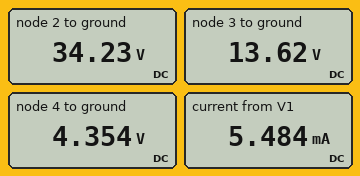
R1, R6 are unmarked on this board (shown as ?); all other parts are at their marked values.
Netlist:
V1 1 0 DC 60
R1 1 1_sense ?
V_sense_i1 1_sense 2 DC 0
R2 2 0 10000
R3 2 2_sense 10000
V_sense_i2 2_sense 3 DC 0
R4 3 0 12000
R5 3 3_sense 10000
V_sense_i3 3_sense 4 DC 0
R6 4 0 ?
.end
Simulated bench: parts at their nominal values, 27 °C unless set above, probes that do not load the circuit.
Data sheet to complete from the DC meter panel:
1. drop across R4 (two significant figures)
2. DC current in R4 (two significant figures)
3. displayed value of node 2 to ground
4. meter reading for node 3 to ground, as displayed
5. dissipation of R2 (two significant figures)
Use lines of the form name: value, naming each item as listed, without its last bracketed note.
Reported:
drop across R4: 14 V
DC current in R4: 1.1 mA
displayed value of node 2 to ground: 34.23 V
meter reading for node 3 to ground, as displayed: 13.62 V
dissipation of R2: 120 mW
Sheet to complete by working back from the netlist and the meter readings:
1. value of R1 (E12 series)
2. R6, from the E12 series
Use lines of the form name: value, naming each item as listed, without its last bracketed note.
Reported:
value of R1: 4.7 kΩ
R6, from the E12 series: 4.7 kΩ
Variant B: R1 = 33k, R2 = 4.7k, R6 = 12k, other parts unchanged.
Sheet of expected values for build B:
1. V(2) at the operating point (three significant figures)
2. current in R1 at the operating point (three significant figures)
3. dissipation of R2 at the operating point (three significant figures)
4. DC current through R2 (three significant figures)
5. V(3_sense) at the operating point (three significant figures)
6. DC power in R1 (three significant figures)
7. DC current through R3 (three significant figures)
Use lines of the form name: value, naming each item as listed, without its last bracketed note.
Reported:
V(2) at the operating point: 6.07 V
current in R1 at the operating point: 1.63 mA
dissipation of R2 at the operating point: 7.85 mW
DC current through R2: 1.29 mA
V(3_sense) at the operating point: 1.45 V
DC power in R1: 88.1 mW
DC current through R3: 342 µA
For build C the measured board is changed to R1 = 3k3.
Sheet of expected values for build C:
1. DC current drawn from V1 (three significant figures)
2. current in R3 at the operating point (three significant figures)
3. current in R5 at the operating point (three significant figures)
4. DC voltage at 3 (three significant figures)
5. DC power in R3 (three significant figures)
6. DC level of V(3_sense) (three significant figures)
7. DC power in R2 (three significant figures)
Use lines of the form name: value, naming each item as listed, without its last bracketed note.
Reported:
DC current drawn from V1: 6.29 mA
current in R3 at the operating point: 2.36 mA
current in R5 at the operating point: 1.06 mA
DC voltage at 3: 15.6 V
DC power in R3: 55.9 mW
DC level of V(3_sense): 4.99 V
DC power in R2: 154 mW
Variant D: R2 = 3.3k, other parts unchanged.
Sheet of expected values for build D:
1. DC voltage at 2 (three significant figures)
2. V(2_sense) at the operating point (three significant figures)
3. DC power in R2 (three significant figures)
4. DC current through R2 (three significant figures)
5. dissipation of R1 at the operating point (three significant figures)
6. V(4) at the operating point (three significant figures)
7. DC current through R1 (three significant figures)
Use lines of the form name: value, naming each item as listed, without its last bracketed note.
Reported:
DC voltage at 2: 22.2 V
V(2_sense) at the operating point: 8.82 V
DC power in R2: 149 mW
DC current through R2: 6.72 mA
dissipation of R1 at the operating point: 305 mW
V(4) at the operating point: 2.82 V
DC current through R1: 8.05 mA
